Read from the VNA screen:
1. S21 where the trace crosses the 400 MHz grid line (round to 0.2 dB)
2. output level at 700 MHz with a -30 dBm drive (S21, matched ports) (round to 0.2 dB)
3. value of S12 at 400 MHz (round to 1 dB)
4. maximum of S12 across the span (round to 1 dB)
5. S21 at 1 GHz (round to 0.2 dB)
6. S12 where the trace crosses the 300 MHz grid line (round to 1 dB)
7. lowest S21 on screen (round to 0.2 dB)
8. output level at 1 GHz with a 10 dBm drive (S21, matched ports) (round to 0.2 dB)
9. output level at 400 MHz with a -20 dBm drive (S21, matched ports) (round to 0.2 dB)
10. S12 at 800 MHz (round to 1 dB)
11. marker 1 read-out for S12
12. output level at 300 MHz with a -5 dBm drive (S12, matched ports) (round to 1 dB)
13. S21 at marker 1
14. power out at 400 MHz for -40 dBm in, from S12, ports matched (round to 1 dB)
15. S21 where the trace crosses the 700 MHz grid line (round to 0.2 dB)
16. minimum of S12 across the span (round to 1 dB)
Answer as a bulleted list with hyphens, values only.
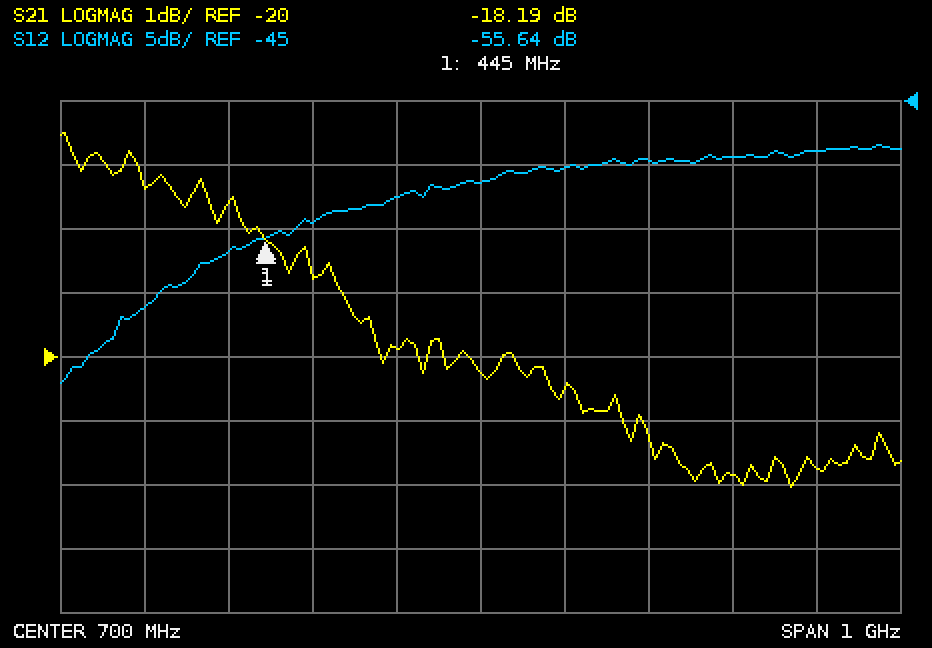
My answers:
- -17.6 dB
- -50.2 dBm
- -57 dB
- -48 dB
- -21.8 dB
- -61 dB
- -22.0 dB
- -11.8 dBm
- -37.6 dBm
- -50 dB
- -55.64 dB
- -66 dBm
- -18.19 dB
- -97 dBm
- -20.2 dB
- -67 dB
